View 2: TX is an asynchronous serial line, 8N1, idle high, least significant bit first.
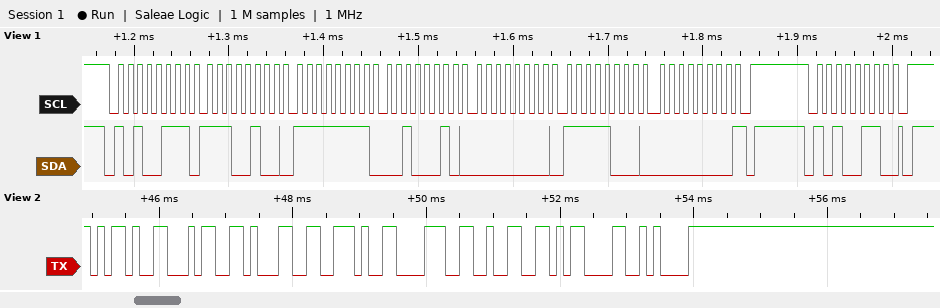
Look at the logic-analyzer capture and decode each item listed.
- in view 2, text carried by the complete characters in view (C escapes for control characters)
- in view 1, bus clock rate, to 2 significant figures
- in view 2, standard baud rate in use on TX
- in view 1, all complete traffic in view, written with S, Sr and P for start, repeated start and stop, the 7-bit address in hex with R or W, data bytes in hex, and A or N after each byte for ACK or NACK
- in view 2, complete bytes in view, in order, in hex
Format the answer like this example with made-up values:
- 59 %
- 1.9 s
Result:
- "-41.82\r\n"
- 100 kHz
- 9600 baud
- S 53R A E4 A FF A 22 A 00 A F8 A 00 N P S 53W A P
- 2D 34 31 2E 38 32 0D 0A
